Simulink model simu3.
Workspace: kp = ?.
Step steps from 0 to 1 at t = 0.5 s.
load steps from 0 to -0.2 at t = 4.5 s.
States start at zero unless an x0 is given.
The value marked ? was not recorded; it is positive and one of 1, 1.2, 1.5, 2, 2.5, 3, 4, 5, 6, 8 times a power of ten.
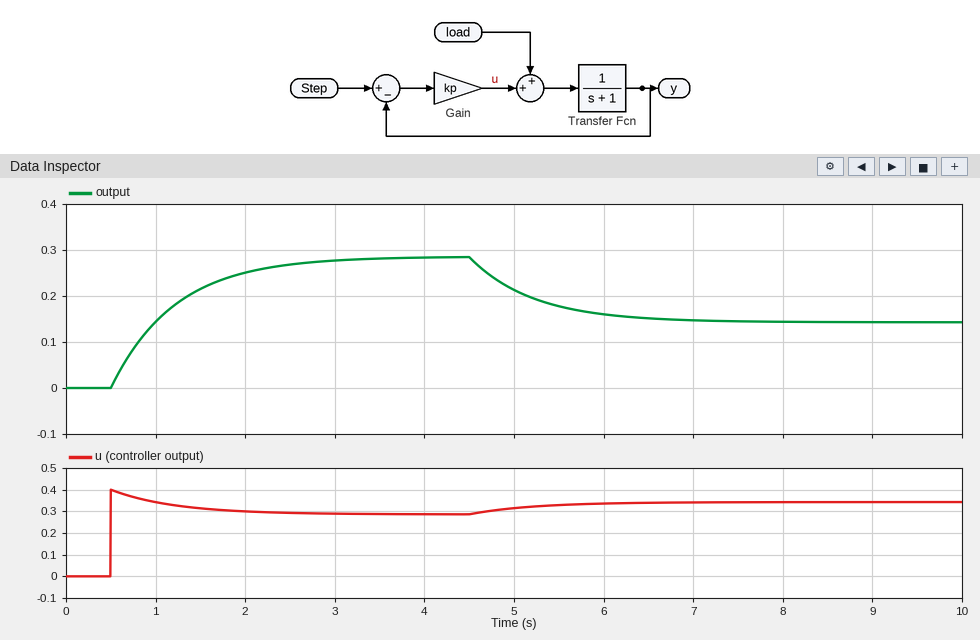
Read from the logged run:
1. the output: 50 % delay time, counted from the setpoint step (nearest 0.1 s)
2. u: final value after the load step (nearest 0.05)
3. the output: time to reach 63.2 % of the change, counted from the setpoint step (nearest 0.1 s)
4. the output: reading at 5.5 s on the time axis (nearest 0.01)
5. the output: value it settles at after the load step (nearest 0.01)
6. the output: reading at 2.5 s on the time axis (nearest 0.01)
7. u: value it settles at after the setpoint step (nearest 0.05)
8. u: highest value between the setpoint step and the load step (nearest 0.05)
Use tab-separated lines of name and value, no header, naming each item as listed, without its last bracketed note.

the output: 50 % delay time, counted from the setpoint step	0.5 s
u: final value after the load step	0.35
the output: time to reach 63.2 % of the change, counted from the setpoint step	0.7 s
the output: reading at 5.5 s on the time axis	0.18
the output: value it settles at after the load step	0.14
the output: reading at 2.5 s on the time axis	0.27
u: value it settles at after the setpoint step	0.30
u: highest value between the setpoint step and the load step	0.40
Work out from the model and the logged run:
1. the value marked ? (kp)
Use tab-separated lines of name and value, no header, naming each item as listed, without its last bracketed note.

the value marked ?	0.4
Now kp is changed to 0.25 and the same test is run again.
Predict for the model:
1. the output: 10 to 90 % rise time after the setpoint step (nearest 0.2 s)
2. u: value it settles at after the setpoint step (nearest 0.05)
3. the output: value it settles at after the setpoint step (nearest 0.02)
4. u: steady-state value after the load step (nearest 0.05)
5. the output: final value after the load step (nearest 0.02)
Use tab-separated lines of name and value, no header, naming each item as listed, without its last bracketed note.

the output: 10 to 90 % rise time after the setpoint step	1.8 s
u: value it settles at after the setpoint step	0.20
the output: value it settles at after the setpoint step	0.20
u: steady-state value after the load step	0.25
the output: final value after the load step	0.04
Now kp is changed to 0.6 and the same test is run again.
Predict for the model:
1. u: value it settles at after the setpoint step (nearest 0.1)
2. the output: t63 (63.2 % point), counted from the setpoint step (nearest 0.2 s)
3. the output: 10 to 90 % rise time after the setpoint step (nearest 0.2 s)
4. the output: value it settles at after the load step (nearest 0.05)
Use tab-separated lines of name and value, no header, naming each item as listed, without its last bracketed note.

u: value it settles at after the setpoint step	0.4
the output: t63 (63.2 % point), counted from the setpoint step	0.6 s
the output: 10 to 90 % rise time after the setpoint step	1.4 s
the output: value it settles at after the load step	0.25
